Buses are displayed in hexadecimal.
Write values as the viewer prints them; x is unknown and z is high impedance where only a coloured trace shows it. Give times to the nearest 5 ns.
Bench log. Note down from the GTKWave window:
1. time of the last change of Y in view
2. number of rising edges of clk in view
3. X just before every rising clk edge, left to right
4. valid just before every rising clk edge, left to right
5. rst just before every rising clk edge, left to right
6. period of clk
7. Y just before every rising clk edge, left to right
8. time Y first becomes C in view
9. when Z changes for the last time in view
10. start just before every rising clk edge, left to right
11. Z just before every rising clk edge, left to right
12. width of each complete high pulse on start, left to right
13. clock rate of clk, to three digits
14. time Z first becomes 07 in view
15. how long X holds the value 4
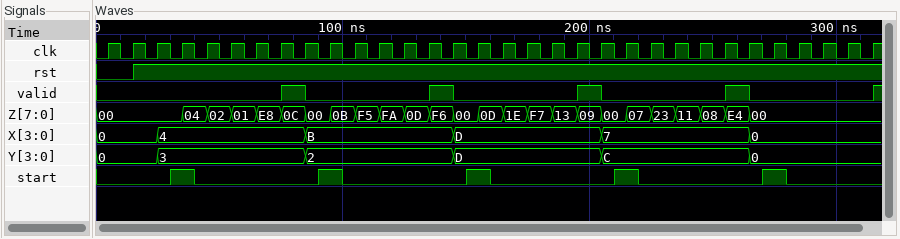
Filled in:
265 ns
32
0, 0, 0, 4, 4, 4, 4, 4, 4, B, B, B, B, B, B, D, D, D, D, D, D, 7, 7, 7, 7, 7, 7, 0, 0, 0, 0, 0
0 0 0 0 0 0 0 0 1 0 0 0 0 0 1 0 0 0 0 0 1 0 0 0 0 0 1 0 0 0 0 0
0 0 1 1 1 1 1 1 1 1 1 1 1 1 1 1 1 1 1 1 1 1 1 1 1 1 1 1 1 1 1 1
10 ns
0, 0, 0, 3, 3, 3, 3, 3, 3, 2, 2, 2, 2, 2, 2, D, D, D, D, D, D, C, C, C, C, C, C, 0, 0, 0, 0, 0
205 ns
265 ns
0 0 0 1 0 0 0 0 0 1 0 0 0 0 0 1 0 0 0 0 0 1 0 0 0 0 0 1 0 0 0 0
00, 00, 00, 00, 04, 02, 01, E8, 0C, 00, 0B, F5, FA, 0D, F6, 00, 0D, 1E, F7, 13, 09, 00, 07, 23, 11, 08, E4, 00, 00, 00, 00, 00
10 ns, 10 ns, 10 ns, 10 ns, 10 ns
100 MHz
215 ns
60 ns
